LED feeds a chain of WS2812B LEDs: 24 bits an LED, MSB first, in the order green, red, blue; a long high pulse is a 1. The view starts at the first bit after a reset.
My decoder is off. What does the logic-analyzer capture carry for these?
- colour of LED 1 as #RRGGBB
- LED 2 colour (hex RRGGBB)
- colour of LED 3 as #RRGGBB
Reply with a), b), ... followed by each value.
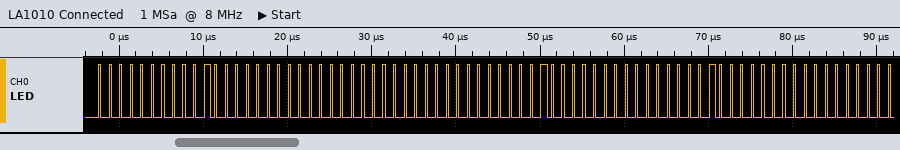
a) #200000
b) #000020
c) #200000
